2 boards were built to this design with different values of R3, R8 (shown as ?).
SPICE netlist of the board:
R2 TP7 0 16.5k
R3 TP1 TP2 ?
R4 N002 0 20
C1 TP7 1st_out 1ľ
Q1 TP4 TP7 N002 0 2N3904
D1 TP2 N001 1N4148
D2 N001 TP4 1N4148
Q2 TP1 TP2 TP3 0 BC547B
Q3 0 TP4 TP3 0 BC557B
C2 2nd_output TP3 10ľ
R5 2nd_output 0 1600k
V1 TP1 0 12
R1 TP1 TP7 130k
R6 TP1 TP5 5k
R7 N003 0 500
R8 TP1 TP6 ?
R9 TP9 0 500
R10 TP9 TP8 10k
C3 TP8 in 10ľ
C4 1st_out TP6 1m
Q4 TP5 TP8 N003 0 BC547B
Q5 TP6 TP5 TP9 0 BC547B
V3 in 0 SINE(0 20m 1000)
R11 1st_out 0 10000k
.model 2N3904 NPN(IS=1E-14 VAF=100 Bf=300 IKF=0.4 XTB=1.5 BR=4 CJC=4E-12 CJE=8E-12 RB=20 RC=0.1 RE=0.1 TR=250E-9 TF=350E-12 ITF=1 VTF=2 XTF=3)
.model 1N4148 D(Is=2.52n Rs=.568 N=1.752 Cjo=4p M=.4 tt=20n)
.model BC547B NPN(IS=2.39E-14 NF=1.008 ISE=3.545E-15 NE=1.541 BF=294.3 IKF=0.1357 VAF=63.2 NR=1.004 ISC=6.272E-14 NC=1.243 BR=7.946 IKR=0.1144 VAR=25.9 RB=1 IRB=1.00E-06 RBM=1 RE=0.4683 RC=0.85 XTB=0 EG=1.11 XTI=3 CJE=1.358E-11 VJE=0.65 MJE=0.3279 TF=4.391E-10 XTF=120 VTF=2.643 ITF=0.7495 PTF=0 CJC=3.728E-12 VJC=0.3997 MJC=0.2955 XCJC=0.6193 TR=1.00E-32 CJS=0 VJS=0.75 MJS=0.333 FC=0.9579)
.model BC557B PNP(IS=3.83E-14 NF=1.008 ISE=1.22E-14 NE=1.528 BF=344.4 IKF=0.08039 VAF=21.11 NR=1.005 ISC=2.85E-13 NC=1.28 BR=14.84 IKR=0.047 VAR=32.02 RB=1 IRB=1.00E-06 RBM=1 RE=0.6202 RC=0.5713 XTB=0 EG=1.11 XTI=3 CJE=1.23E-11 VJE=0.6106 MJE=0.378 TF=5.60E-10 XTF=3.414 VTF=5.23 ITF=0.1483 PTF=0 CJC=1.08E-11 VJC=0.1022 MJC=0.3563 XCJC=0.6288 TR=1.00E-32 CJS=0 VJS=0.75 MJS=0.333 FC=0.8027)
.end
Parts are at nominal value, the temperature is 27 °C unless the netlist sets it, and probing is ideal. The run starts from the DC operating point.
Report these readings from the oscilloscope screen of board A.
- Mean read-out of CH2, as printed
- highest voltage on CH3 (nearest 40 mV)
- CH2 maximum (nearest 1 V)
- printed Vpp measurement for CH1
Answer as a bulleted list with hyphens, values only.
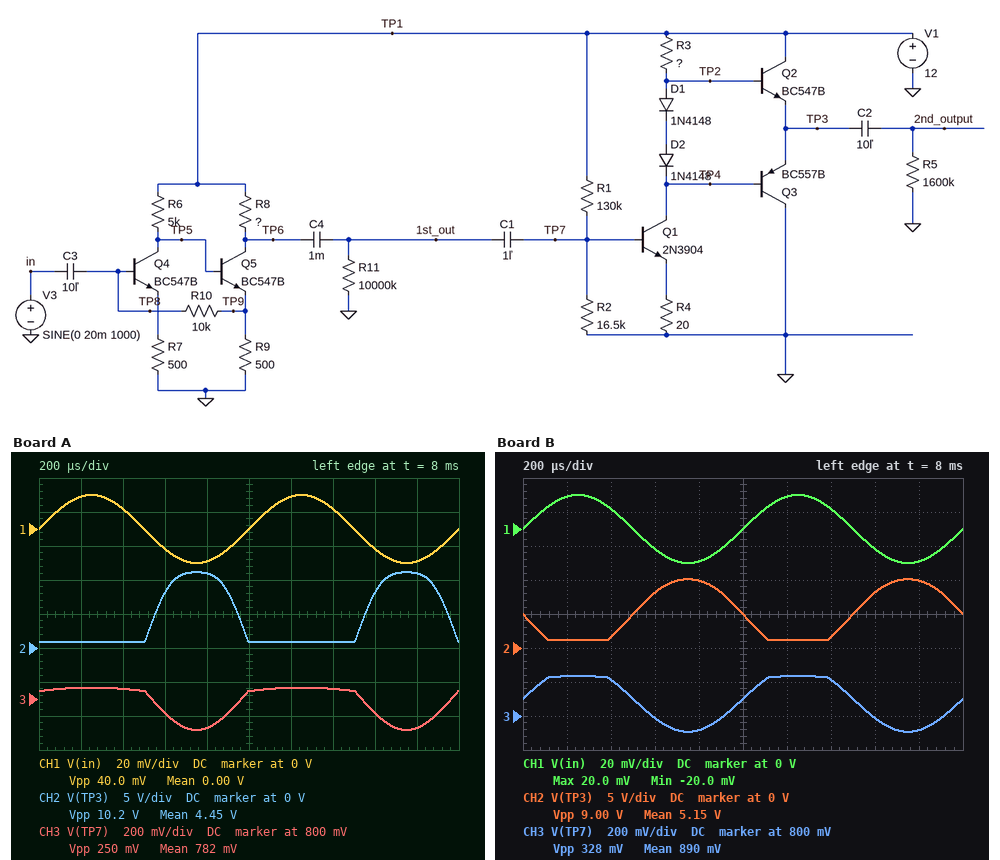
- 4.45 V
- 880 mV
- 11 V
- 40.0 mV
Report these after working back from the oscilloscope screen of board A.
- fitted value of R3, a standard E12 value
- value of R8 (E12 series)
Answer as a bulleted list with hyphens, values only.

- 1.5 kΩ
- 680 Ω
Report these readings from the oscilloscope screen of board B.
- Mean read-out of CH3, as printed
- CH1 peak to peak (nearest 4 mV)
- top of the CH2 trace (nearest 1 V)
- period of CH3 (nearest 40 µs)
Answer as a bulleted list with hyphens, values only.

- 890 mV
- 40 mV
- 10 V
- 1.00 ms
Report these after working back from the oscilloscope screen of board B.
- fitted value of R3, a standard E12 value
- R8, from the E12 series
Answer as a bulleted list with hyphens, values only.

- 680 Ω
- 560 Ω
